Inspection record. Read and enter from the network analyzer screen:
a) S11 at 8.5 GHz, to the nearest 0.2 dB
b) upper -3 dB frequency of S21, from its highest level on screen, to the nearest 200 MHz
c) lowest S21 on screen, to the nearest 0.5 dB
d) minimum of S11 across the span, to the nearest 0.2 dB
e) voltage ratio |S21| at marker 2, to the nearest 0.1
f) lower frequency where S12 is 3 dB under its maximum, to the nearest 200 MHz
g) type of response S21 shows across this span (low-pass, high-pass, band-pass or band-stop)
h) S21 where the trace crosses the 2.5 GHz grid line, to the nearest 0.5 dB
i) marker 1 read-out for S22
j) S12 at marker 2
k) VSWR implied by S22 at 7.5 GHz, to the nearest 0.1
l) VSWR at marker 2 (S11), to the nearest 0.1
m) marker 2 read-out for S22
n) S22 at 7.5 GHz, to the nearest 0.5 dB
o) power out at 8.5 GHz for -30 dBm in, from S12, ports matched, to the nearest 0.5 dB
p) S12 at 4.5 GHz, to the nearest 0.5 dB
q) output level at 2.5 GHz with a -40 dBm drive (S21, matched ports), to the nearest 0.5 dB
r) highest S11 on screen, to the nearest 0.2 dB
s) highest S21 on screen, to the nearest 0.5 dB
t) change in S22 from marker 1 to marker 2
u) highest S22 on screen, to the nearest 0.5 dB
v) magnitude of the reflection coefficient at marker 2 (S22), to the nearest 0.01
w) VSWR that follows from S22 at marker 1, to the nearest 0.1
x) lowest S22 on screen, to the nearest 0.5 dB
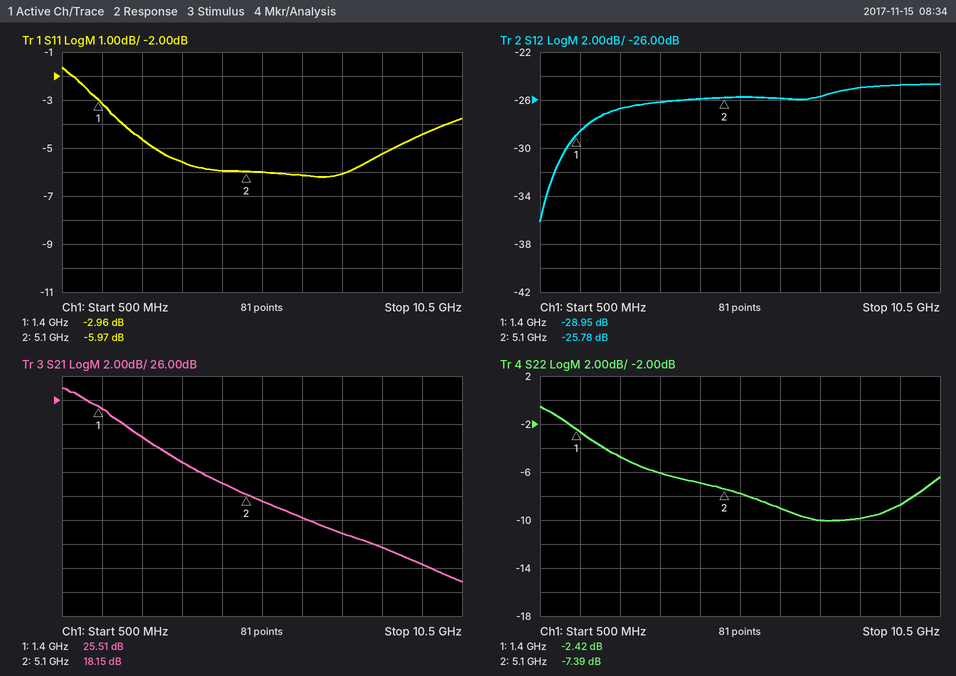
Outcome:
-5.2 dB
2.0 GHz
11.0 dB
-6.2 dB
8.1
1.8 GHz
low-pass
23.0 dB
-2.42 dB
-25.78 dB
1.9
3.0
-7.39 dB
-10.0 dB
-55.0 dBm
-26.0 dB
-17.0 dBm
-1.6 dB
27.0 dB
-4.97 dB
-0.5 dB
0.43
7.2
-10.0 dB
